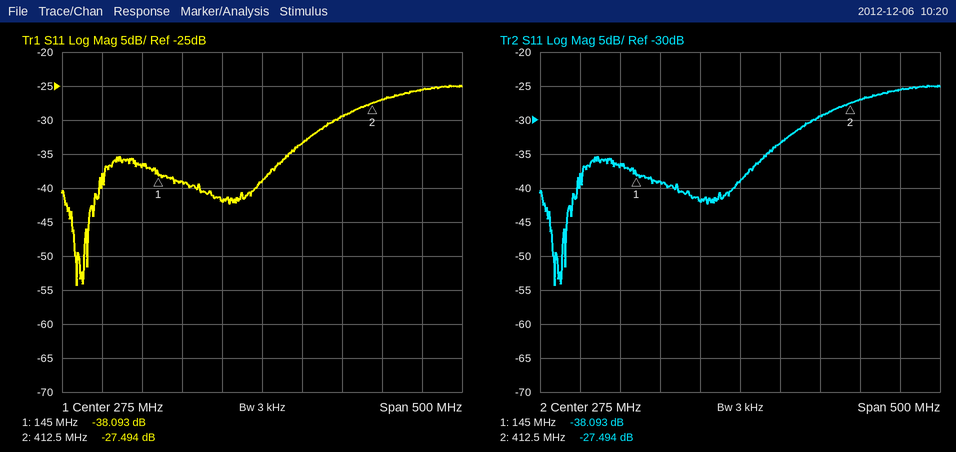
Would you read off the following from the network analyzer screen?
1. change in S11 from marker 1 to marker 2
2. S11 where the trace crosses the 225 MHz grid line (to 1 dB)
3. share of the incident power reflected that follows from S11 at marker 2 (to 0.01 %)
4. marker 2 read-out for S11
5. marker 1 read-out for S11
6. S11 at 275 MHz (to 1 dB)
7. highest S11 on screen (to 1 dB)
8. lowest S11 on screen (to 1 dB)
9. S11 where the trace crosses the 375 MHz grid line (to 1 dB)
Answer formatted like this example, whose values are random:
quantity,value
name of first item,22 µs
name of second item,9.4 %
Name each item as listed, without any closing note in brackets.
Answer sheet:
quantity,value
change in S11 from marker 1 to marker 2,10.599 dB
S11 where the trace crosses the 225 MHz grid line,-42 dB
share of the incident power reflected that follows from S11 at marker 2,0.18 %
marker 2 read-out for S11,-27.494 dB
marker 1 read-out for S11,-38.093 dB
S11 at 275 MHz,-39 dB
highest S11 on screen,-25 dB
lowest S11 on screen,-54 dB
S11 where the trace crosses the 375 MHz grid line,-29 dB
